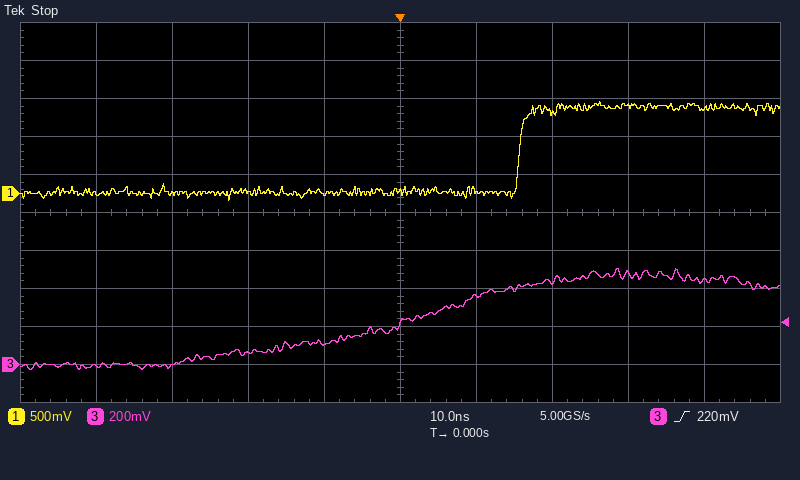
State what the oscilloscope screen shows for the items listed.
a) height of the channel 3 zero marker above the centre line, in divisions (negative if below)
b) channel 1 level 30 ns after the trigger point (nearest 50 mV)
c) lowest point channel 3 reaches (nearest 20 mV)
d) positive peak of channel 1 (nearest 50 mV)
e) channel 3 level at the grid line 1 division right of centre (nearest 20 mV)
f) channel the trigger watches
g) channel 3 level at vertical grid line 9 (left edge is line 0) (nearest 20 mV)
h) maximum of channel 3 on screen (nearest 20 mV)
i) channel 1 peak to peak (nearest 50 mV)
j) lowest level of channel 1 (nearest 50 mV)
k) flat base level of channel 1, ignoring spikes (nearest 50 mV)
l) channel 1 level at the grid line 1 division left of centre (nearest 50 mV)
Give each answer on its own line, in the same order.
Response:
-4.0 div
1.15 V
-20 mV
1.20 V
360 mV
channel 3
440 mV
500 mV
1.30 V
-100 mV
0 mV
0 mV
